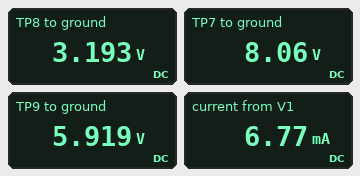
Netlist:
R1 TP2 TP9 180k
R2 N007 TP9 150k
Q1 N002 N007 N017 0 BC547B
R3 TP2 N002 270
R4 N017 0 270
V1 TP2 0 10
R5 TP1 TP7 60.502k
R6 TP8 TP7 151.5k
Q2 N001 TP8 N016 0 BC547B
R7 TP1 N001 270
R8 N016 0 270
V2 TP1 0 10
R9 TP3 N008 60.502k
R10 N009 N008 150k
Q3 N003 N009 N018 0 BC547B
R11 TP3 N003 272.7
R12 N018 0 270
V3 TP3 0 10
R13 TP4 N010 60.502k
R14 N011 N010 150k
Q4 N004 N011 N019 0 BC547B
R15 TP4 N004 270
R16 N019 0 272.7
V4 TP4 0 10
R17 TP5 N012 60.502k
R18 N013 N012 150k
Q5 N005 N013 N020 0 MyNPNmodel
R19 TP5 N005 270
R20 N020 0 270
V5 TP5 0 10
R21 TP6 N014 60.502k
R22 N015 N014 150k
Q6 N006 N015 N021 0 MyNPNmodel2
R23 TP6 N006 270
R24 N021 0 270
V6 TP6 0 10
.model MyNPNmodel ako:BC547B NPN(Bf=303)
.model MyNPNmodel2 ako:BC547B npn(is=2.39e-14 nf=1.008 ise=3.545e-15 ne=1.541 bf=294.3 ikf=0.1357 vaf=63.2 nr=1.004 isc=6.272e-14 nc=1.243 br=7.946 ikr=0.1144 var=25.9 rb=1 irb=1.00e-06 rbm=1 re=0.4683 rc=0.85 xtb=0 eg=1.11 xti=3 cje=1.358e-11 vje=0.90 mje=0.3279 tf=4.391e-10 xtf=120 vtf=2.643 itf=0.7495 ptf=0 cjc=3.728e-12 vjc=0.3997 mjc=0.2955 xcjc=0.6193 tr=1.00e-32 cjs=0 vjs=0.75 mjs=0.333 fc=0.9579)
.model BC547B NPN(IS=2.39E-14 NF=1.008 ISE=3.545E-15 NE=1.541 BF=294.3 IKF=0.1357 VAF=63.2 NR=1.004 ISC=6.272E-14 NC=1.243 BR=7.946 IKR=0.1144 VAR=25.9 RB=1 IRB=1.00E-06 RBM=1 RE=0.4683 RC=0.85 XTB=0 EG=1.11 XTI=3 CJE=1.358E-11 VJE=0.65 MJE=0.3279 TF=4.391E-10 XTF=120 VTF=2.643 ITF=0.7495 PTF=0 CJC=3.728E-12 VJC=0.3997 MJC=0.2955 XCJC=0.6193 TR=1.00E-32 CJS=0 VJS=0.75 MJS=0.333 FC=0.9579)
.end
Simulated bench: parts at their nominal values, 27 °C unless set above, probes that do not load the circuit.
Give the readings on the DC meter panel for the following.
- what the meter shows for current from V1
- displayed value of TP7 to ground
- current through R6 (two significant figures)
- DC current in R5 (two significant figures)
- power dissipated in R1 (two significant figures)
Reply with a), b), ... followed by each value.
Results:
a) 6.77 mA
b) 8.06 V
c) 32 µA
d) 32 µA
e) 93 µW
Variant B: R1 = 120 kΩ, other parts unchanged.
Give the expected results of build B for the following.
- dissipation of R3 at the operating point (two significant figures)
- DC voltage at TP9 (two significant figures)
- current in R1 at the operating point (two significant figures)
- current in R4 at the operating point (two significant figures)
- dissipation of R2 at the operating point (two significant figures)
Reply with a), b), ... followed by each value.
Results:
a) 16 mW
b) 6.8 V
c) 27 µA
d) 7.8 mA
e) 110 µW
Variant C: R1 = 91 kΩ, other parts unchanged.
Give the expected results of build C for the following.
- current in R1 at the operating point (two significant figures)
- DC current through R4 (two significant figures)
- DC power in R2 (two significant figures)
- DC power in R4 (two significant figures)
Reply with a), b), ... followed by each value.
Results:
a) 29 µA
b) 8.5 mA
c) 130 µW
d) 19 mW
